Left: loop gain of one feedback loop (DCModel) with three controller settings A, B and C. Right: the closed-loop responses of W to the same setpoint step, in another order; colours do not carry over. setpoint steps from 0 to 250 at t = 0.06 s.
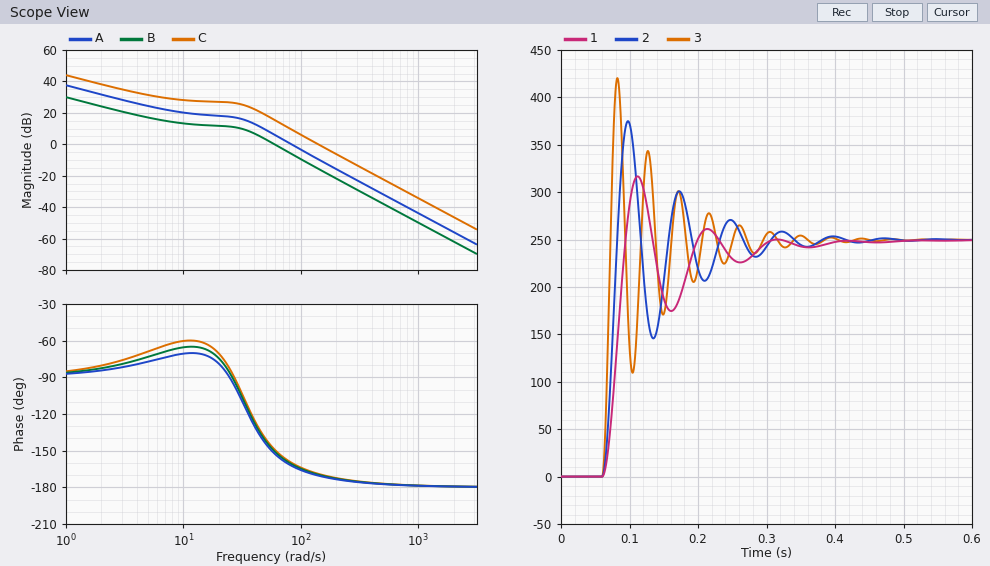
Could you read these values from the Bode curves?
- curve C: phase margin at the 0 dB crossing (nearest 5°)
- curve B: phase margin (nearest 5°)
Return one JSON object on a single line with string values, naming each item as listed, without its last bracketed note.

{"curve C: phase margin at the 0 dB crossing": "10°", "curve B: phase margin": "30°"}
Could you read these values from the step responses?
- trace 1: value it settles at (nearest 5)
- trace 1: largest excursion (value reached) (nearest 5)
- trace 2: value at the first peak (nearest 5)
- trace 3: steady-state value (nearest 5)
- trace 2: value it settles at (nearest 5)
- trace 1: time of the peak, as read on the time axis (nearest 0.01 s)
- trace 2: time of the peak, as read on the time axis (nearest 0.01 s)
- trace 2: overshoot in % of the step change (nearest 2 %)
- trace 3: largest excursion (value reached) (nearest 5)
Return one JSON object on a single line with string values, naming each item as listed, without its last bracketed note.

{"trace 1: value it settles at": "250", "trace 1: largest excursion (value reached)": "315", "trace 2: value at the first peak": "375", "trace 3: steady-state value": "250", "trace 2: value it settles at": "250", "trace 1: time of the peak, as read on the time axis": "0.11 s", "trace 2: time of the peak, as read on the time axis": "0.10 s", "trace 2: overshoot in % of the step change": "50 %", "trace 3: largest excursion (value reached)": "420"}
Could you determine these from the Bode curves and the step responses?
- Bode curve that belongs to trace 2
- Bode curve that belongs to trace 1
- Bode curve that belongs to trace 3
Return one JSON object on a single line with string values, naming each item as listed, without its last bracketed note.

{"Bode curve that belongs to trace 2": "A", "Bode curve that belongs to trace 1": "B", "Bode curve that belongs to trace 3": "C"}
